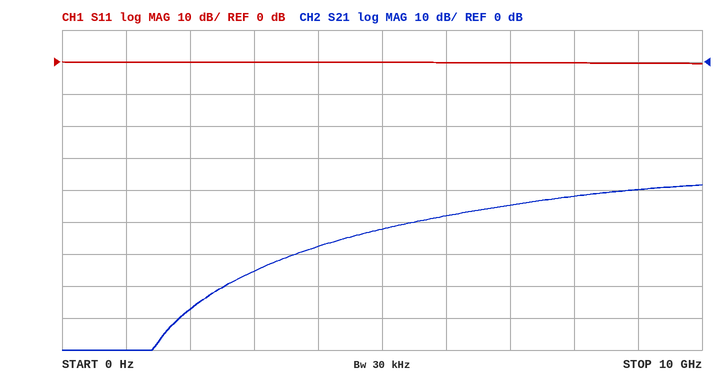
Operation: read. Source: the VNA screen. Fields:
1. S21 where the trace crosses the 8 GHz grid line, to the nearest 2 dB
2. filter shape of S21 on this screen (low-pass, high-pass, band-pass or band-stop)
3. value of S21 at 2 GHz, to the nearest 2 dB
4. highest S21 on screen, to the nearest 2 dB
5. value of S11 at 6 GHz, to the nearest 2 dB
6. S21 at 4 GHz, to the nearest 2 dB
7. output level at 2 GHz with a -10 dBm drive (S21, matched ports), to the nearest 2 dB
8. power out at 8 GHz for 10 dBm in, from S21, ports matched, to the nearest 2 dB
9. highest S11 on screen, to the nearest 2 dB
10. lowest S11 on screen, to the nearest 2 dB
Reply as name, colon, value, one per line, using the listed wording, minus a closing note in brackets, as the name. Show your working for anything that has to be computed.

S21 where the trace crosses the 8 GHz grid line, to the nearest 2 dB: -42 dB
filter shape of S21 on this screen: high-pass
value of S21 at 2 GHz, to the nearest 2 dB: -78 dB
highest S21 on screen, to the nearest 2 dB: -38 dB
value of S11 at 6 GHz, to the nearest 2 dB: 0 dB
S21 at 4 GHz, to the nearest 2 dB: -58 dB
output level at 2 GHz with a -10 dBm drive (S21, matched ports), to the nearest 2 dB: -10 dBm + (-78 dB) = -88 dBm
power out at 8 GHz for 10 dBm in, from S21, ports matched, to the nearest 2 dB: 10 dBm + (-42 dB) = -32 dBm
highest S11 on screen, to the nearest 2 dB: 0 dB
lowest S11 on screen, to the nearest 2 dB: 0 dB
